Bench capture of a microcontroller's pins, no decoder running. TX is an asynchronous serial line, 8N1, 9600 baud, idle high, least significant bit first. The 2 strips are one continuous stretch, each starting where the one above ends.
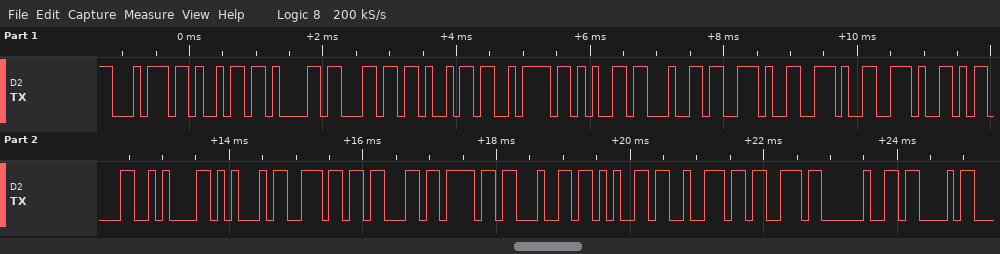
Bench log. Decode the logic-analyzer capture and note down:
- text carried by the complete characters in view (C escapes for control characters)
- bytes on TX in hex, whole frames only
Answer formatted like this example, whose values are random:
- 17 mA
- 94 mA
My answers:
- "tialized...\r\nEncoders C"
- 74 69 61 6C 69 7A 65 64 2E 2E 2E 0D 0A 45 6E 63 6F 64 65 72 73 20 43
